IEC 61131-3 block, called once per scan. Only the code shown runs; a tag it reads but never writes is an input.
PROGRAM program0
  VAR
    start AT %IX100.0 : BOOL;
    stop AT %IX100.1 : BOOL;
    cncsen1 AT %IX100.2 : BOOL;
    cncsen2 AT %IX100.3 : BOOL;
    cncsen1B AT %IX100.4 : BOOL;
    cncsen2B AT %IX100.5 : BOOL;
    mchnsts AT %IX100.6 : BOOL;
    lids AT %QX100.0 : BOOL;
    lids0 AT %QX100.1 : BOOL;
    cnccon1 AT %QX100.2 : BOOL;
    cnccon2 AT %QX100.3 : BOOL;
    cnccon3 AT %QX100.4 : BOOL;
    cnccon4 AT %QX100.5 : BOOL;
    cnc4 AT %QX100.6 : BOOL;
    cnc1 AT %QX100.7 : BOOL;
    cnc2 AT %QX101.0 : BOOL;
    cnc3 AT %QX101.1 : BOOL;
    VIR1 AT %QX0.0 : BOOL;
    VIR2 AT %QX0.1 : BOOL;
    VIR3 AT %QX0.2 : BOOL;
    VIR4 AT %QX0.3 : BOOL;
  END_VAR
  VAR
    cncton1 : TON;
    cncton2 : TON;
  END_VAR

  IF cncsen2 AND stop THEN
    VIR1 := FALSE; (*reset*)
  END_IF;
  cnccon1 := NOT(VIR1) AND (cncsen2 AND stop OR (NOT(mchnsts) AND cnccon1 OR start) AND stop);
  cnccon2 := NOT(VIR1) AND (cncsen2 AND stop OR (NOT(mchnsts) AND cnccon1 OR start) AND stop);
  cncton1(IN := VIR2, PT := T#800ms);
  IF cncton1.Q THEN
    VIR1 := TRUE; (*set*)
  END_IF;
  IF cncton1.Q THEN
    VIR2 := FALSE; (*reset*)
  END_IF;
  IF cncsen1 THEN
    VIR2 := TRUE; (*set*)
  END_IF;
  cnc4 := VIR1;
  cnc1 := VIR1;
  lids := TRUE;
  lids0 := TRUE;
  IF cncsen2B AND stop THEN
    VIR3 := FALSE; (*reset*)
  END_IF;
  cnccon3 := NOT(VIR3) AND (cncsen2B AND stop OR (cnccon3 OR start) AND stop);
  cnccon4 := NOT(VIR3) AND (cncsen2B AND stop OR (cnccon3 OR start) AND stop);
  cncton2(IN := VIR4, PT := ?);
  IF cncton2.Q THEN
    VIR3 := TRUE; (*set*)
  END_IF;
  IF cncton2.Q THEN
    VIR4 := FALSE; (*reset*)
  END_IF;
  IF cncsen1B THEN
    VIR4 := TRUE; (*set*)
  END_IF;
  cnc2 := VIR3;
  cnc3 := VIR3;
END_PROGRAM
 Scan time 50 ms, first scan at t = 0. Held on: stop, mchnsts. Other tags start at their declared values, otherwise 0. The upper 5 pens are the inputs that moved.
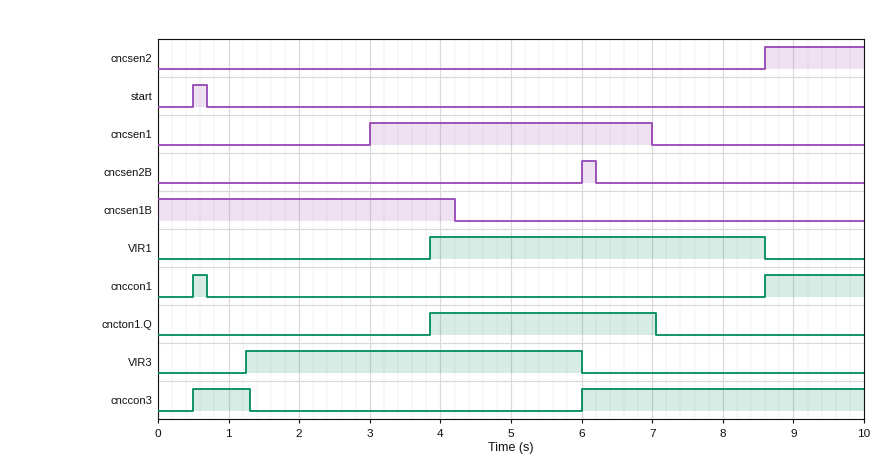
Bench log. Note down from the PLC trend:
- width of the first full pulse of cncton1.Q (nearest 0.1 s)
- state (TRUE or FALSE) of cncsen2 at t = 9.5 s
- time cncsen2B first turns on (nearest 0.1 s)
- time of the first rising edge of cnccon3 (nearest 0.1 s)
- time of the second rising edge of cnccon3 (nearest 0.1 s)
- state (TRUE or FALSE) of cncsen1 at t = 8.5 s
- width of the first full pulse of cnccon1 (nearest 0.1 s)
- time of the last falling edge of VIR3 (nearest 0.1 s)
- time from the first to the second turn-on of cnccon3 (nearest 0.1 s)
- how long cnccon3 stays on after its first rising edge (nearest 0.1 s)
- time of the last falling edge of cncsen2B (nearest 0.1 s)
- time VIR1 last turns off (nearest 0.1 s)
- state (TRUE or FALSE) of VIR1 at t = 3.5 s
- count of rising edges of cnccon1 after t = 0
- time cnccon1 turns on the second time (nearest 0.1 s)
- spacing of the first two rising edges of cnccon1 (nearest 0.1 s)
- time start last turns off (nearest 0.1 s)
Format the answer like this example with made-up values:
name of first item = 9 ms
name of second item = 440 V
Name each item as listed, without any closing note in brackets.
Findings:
width of the first full pulse of cncton1.Q = 3.2 s
state (TRUE or FALSE) of cncsen2 at t = 9.5 s = TRUE
time cncsen2B first turns on = 6.0 s
time of the first rising edge of cnccon3 = 0.5 s
time of the second rising edge of cnccon3 = 6.0 s
state (TRUE or FALSE) of cncsen1 at t = 8.5 s = FALSE
width of the first full pulse of cnccon1 = 0.2 s
time of the last falling edge of VIR3 = 6.0 s
time from the first to the second turn-on of cnccon3 = 5.5 s
how long cnccon3 stays on after its first rising edge = 0.8 s
time of the last falling edge of cncsen2B = 6.2 s
time VIR1 last turns off = 8.6 s
state (TRUE or FALSE) of VIR1 at t = 3.5 s = FALSE
count of rising edges of cnccon1 after t = 0 = 2
time cnccon1 turns on the second time = 8.6 s
spacing of the first two rising edges of cnccon1 = 8.1 s
time start last turns off = 0.7 s
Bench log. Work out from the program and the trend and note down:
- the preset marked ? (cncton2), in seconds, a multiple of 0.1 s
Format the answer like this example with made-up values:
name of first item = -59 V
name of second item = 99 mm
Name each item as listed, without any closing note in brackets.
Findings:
the preset marked ? (cncton2), in seconds, a multiple of 0.1 s = 1.2 s
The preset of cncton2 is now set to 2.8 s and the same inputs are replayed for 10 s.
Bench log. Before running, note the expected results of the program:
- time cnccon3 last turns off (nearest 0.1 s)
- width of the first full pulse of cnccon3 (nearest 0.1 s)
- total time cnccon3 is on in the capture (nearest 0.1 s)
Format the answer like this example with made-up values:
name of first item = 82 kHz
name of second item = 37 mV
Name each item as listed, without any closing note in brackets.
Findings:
time cnccon3 last turns off = 2.9 s
width of the first full pulse of cnccon3 = 2.4 s
total time cnccon3 is on in the capture = 6.4 s
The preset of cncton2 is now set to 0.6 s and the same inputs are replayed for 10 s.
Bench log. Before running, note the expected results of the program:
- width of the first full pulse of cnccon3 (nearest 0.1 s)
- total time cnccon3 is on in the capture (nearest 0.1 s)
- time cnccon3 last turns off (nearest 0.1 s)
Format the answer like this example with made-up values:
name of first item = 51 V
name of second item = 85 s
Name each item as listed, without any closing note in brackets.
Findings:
width of the first full pulse of cnccon3 = 0.2 s
total time cnccon3 is on in the capture = 4.2 s
time cnccon3 last turns off = 0.7 s
